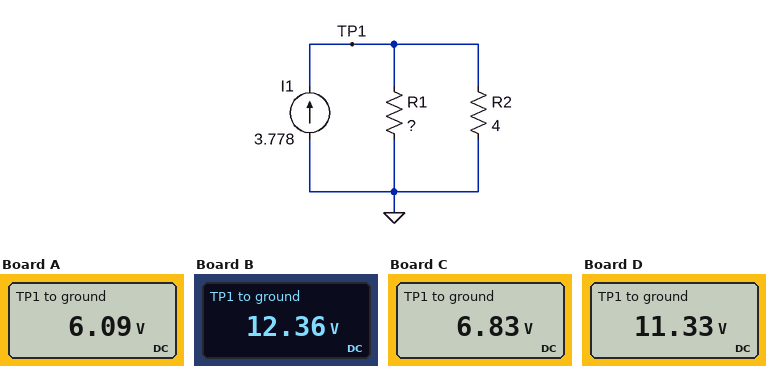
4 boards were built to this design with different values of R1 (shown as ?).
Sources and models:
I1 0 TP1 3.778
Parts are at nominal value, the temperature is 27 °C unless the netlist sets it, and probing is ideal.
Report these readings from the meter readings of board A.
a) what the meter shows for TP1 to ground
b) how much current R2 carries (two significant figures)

6.09 V
1.5 A
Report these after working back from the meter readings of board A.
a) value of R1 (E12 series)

2.7 Ω
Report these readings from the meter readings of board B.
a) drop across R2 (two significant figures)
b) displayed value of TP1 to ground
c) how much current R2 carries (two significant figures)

12 V
12.36 V
3.1 A
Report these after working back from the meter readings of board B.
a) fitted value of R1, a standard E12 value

18 Ω
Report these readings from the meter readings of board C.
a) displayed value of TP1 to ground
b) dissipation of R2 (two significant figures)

6.83 V
12 W
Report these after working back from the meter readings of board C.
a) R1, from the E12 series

3.3 Ω
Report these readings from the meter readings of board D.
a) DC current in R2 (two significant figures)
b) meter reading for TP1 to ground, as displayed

2.8 A
11.33 V
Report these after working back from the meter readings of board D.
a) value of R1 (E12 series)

12 Ω
